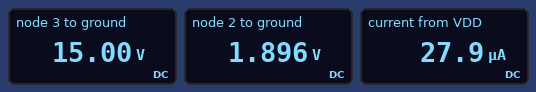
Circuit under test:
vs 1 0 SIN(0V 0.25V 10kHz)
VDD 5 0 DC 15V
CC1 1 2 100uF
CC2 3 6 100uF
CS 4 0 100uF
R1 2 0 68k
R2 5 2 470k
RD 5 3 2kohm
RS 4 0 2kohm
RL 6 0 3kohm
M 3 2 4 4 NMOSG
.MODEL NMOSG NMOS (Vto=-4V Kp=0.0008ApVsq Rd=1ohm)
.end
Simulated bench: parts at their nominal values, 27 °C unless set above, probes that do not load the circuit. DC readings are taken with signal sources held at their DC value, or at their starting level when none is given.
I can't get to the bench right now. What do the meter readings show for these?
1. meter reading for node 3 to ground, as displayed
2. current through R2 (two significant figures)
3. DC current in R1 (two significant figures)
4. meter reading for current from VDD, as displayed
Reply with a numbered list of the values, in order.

1. 15.00 V
2. 28 µA
3. 28 µA
4. 27.9 µA
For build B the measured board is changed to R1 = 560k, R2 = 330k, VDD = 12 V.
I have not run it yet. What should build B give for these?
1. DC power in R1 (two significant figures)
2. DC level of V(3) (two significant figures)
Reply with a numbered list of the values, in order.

1. 100 µW
2. 12 V
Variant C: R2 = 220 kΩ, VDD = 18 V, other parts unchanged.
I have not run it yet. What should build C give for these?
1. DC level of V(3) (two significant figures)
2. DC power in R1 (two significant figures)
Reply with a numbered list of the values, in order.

1. 18 V
2. 270 µW
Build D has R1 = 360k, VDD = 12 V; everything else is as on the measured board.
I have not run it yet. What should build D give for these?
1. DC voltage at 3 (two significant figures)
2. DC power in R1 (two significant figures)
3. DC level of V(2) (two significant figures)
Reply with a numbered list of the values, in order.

1. 12 V
2. 75 µW
3. 5.2 V
